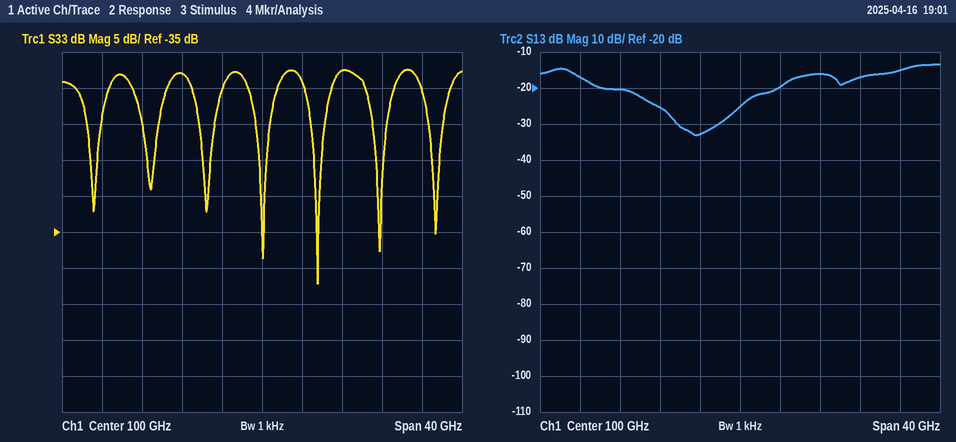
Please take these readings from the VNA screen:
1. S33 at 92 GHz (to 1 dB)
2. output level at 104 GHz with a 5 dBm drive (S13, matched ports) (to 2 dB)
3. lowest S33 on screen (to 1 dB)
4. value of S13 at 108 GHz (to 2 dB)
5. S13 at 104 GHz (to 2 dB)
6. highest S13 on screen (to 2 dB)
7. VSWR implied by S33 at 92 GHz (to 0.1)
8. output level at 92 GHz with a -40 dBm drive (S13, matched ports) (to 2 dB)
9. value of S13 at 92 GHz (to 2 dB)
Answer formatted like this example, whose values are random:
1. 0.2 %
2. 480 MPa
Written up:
1. -13 dB
2. -14 dBm
3. -42 dB
4. -16 dB
5. -20 dB
6. -14 dB
7. 1.6
8. -66 dBm
9. -26 dB
